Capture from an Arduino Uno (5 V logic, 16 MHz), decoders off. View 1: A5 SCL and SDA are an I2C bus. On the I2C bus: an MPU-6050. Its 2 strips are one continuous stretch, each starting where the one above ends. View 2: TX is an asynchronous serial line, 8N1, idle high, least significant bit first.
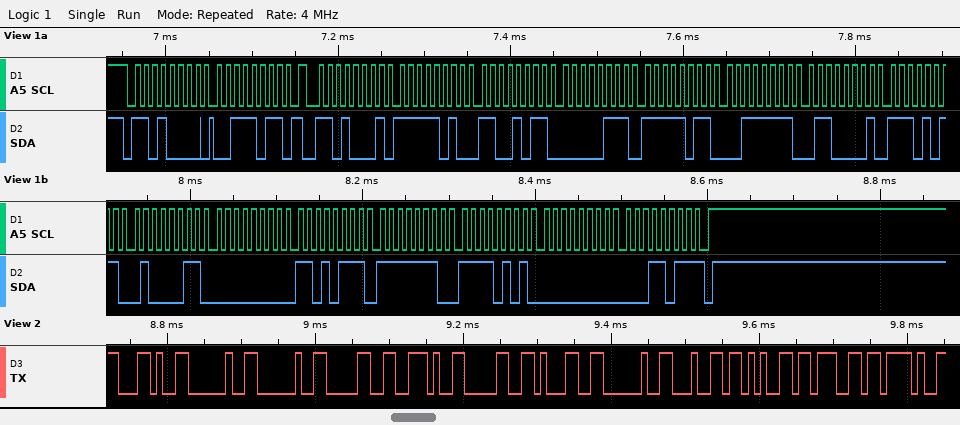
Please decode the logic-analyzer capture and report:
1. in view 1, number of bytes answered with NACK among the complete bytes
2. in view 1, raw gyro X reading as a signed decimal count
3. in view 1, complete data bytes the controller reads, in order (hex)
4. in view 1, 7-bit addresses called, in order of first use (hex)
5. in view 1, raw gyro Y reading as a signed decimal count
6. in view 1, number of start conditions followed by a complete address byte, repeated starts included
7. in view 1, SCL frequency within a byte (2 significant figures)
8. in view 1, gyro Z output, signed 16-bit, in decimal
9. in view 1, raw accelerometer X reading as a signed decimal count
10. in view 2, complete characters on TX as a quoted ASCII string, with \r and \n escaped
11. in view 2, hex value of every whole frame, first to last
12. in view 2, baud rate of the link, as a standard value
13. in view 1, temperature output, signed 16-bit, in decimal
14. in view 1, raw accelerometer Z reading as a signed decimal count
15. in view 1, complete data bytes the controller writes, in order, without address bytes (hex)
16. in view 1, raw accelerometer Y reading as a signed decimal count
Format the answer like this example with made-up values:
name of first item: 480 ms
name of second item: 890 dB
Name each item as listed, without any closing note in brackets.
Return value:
in view 1, number of bytes answered with NACK among the complete bytes: 1
in view 1, raw gyro X reading as a signed decimal count: 215
in view 1, complete data bytes the controller reads, in order: FA CB 07 FB 3F 61 EB 43 00 D7 FE F5 00 1B
in view 1, 7-bit addresses called, in order of first use: 0x68
in view 1, raw gyro Y reading as a signed decimal count: -267
in view 1, number of start conditions followed by a complete address byte, repeated starts included: 2
in view 1, SCL frequency within a byte: 100 kHz
in view 1, gyro Z output, signed 16-bit, in decimal: 27
in view 1, raw accelerometer X reading as a signed decimal count: -1333
in view 2, complete characters on TX as a quoted ASCII string, with \r and \n escaped: ",  0.01 deg/"
in view 2, hex value of every whole frame, first to last: 2C 20 20 30 2E 30 31 20 64 65 67 2F
in view 2, baud rate of the link, as a standard value: 115200 baud
in view 1, temperature output, signed 16-bit, in decimal: -5309
in view 1, raw accelerometer Z reading as a signed decimal count: 16225
in view 1, complete data bytes the controller writes, in order, without address bytes: 3B
in view 1, raw accelerometer Y reading as a signed decimal count: 2043
